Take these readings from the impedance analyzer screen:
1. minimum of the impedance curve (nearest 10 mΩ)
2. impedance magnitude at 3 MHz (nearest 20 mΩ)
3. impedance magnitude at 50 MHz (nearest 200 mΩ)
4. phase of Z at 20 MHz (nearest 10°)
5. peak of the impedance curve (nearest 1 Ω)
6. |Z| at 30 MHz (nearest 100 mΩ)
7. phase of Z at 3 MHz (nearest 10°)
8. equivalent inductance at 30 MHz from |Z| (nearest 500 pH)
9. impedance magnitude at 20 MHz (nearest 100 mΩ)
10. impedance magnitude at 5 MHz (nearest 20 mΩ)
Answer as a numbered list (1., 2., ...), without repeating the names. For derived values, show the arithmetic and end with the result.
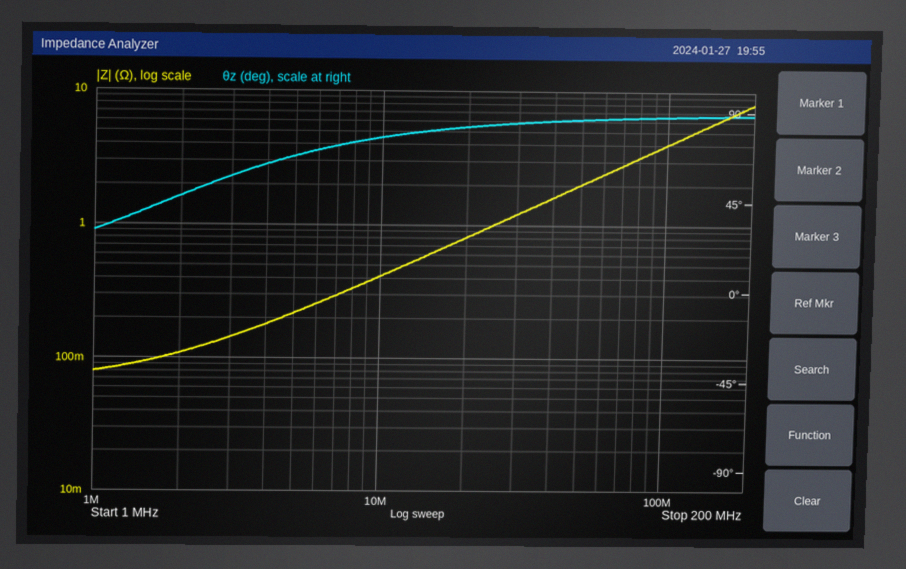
1. 80 mΩ
2. 140 mΩ
3. 2.0 Ω
4. 80°
5. 8 Ω
6. 1.2 Ω
7. 60°
8. L = 1.2 Ω/(2π × 30 MHz) ≈ 6.37 nH, so 6.5 nH to the nearest 500 pH
9. 800 mΩ
10. 220 mΩ
